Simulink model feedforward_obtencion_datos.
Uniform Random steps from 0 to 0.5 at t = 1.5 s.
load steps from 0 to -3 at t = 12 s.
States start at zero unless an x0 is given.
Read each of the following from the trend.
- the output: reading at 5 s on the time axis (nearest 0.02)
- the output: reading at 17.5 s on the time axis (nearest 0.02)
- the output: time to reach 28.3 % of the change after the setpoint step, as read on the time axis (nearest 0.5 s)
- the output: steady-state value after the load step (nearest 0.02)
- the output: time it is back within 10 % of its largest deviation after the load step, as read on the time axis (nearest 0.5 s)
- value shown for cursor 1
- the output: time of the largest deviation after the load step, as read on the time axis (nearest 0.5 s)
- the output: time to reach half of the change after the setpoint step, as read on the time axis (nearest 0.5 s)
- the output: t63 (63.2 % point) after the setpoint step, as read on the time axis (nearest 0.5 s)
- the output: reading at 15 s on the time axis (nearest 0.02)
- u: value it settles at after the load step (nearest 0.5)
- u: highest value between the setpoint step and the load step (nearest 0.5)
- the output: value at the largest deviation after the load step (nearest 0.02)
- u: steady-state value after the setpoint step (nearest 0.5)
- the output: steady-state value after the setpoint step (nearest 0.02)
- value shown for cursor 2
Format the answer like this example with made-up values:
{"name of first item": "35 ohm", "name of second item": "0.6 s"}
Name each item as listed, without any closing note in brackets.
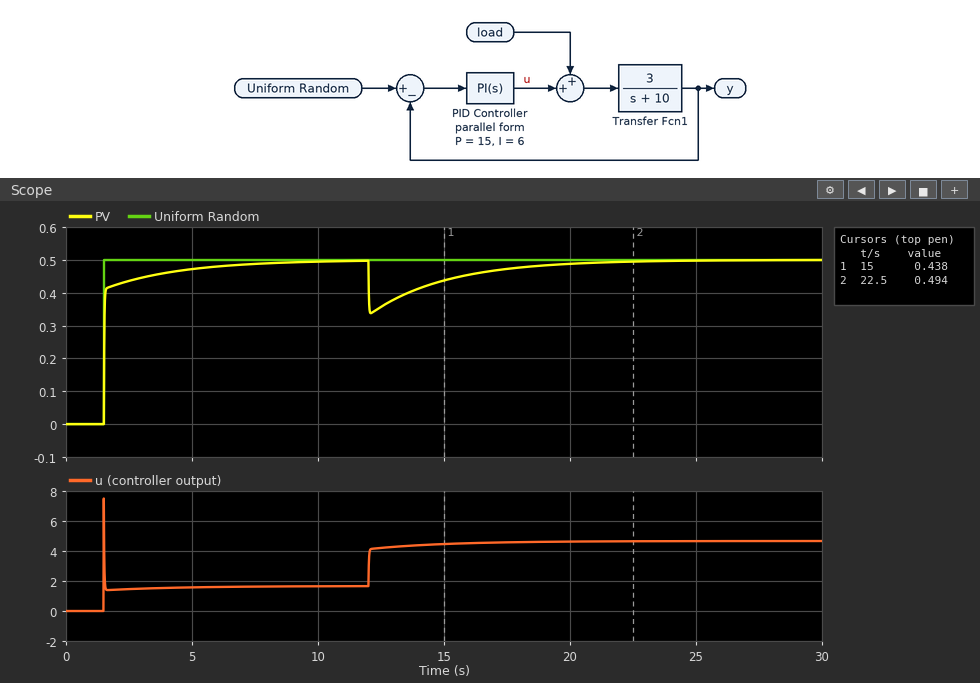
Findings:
{"the output: reading at 5 s on the time axis": "0.48", "the output: reading at 17.5 s on the time axis": "0.48", "the output: time to reach 28.3 % of the change after the setpoint step, as read on the time axis": "1.5 s", "the output: steady-state value after the load step": "0.50", "the output: time it is back within 10 % of its largest deviation after the load step, as read on the time axis": "19.0 s", "value shown for cursor 1": "0.438", "the output: time of the largest deviation after the load step, as read on the time axis": "12.0 s", "the output: time to reach half of the change after the setpoint step, as read on the time axis": "1.5 s", "the output: t63 (63.2 % point) after the setpoint step, as read on the time axis": "1.5 s", "the output: reading at 15 s on the time axis": "0.44", "u: value it settles at after the load step": "4.5", "u: highest value between the setpoint step and the load step": "7.5", "the output: value at the largest deviation after the load step": "0.34", "u: steady-state value after the setpoint step": "1.5", "the output: steady-state value after the setpoint step": "0.50", "value shown for cursor 2": "0.494"}
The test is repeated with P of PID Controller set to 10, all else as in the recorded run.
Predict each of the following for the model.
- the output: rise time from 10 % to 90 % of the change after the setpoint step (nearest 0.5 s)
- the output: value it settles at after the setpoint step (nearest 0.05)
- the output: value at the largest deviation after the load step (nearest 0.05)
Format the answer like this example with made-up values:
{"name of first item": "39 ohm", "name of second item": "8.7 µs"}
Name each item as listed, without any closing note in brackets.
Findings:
{"the output: rise time from 10 % to 90 % of the change after the setpoint step": "2.0 s", "the output: value it settles at after the setpoint step": "0.50", "the output: value at the largest deviation after the load step": "0.30"}
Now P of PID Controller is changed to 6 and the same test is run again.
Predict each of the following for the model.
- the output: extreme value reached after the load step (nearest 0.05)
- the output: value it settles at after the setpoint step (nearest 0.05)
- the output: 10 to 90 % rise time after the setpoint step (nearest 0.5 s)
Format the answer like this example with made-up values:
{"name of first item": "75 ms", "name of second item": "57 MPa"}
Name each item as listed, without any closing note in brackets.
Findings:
{"the output: extreme value reached after the load step": "0.20", "the output: value it settles at after the setpoint step": "0.50", "the output: 10 to 90 % rise time after the setpoint step": "2.0 s"}
